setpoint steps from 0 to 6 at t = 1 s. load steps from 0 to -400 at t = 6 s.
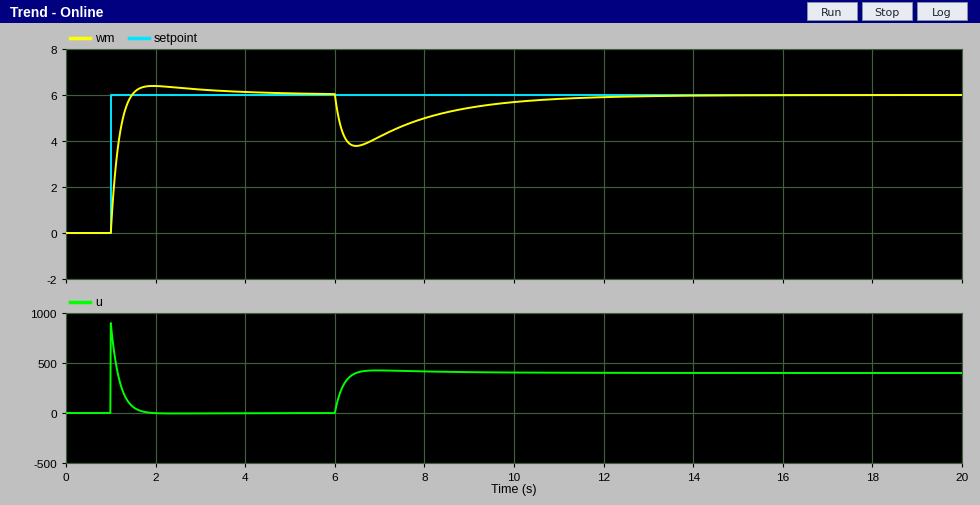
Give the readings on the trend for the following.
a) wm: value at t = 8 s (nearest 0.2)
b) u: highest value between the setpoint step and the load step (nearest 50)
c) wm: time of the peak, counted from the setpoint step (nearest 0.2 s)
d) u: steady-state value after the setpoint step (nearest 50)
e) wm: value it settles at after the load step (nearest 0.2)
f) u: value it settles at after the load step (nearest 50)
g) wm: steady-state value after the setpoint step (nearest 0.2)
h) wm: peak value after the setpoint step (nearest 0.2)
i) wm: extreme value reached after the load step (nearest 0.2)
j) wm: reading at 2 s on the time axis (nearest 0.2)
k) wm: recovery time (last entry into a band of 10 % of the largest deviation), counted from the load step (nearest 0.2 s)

5.0
900
1.0 s
0
6.0
400
6.0
6.4
3.8
6.4
4.6 s
